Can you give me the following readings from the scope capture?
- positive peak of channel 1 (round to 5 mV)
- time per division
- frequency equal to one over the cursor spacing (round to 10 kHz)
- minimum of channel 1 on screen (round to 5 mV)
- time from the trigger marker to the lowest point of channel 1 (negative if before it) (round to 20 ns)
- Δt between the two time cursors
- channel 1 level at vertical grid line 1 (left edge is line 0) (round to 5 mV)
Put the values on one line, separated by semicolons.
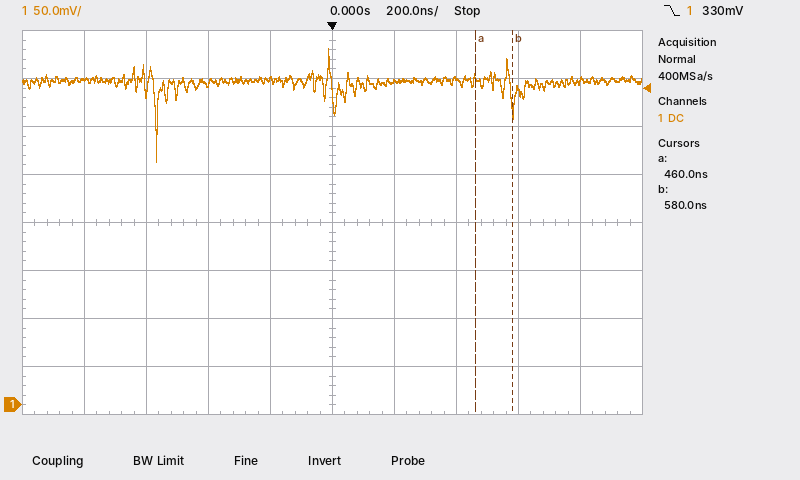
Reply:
370 mV; 200 ns; 8.33 MHz; 255 mV; -560 ns; 120 ns; 340 mV
